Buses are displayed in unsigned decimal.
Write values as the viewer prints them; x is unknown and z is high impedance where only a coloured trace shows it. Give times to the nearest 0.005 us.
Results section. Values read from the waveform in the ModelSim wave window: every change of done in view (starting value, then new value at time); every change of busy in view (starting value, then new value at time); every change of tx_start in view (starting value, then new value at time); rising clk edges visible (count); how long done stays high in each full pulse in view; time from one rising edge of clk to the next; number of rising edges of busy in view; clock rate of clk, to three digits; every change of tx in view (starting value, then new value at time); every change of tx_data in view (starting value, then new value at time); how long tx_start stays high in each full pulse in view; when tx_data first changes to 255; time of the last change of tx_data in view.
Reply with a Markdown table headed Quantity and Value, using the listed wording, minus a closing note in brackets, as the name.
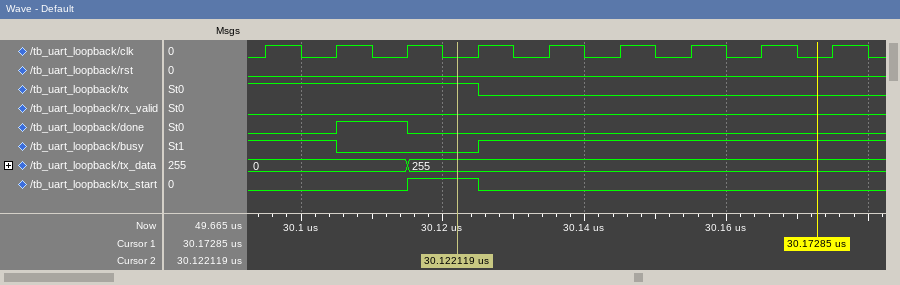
| Quantity | Value |
|---|---|
| every change of done in view | 0, 1 at 30.105 us, 0 at 30.115 us |
| every change of busy in view | 1, 0 at 30.105 us, 1 at 30.125 us |
| every change of tx_start in view | 0, 1 at 30.115 us, 0 at 30.125 us |
| rising clk edges visible | 9 |
| how long done stays high in each full pulse in view | 0.01 us |
| time from one rising edge of clk to the next | 0.01 us |
| number of rising edges of busy in view | 1 |
| clock rate of clk, to three digits | 100 MHz |
| every change of tx in view | 1, 0 at 30.125 us |
| every change of tx_data in view | 0, 255 at 30.115 us |
| how long tx_start stays high in each full pulse in view | 0.01 us |
| when tx_data first changes to 255 | 30.115 us |
| time of the last change of tx_data in view | 30.115 us |
